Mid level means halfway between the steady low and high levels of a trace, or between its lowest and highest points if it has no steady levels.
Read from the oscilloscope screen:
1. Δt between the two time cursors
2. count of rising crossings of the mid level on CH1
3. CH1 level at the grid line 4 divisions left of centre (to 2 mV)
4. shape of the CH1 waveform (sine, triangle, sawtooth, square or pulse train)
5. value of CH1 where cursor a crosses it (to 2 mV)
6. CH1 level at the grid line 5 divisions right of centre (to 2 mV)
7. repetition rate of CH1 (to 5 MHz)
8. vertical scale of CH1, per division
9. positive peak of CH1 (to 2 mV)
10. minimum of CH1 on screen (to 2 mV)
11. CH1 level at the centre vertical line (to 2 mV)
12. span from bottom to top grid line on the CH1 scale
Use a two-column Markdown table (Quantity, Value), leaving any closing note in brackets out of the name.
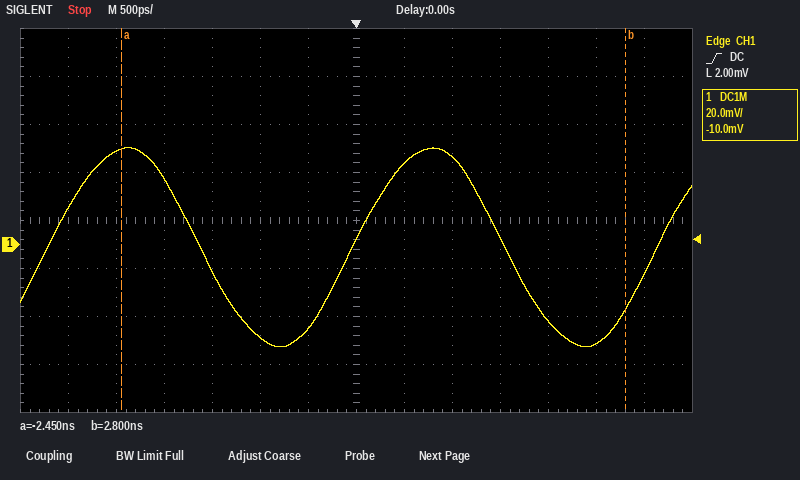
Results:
| Quantity | Value |
|---|---|
| Δt between the two time cursors | 5.25 ns |
| count of rising crossings of the mid level on CH1 | 3 |
| CH1 level at the grid line 4 divisions left of centre | 28 mV |
| shape of the CH1 waveform | sine |
| value of CH1 where cursor a crosses it | 40 mV |
| CH1 level at the grid line 5 divisions right of centre | -42 mV |
| repetition rate of CH1 | 315 MHz |
| vertical scale of CH1, per division | 20 mV |
| positive peak of CH1 | 40 mV |
| minimum of CH1 on screen | -42 mV |
| CH1 level at the centre vertical line | 2 mV |
| span from bottom to top grid line on the CH1 scale | 160 mV |
